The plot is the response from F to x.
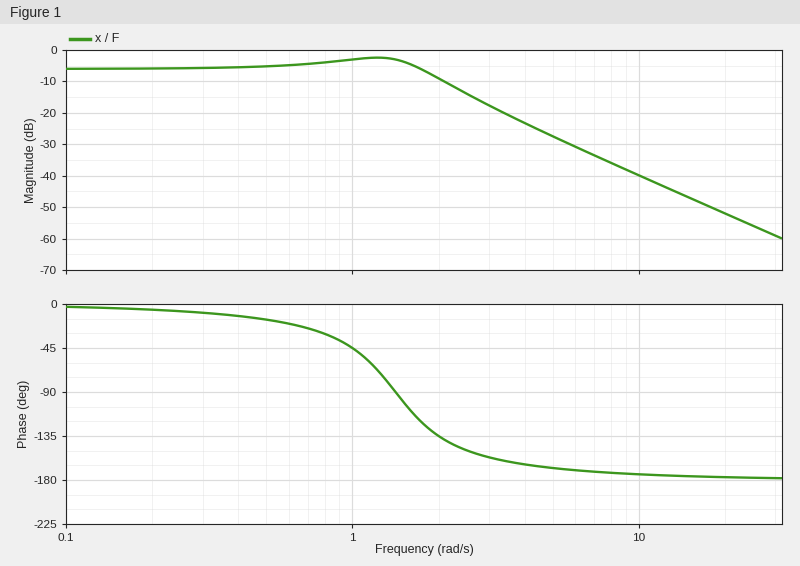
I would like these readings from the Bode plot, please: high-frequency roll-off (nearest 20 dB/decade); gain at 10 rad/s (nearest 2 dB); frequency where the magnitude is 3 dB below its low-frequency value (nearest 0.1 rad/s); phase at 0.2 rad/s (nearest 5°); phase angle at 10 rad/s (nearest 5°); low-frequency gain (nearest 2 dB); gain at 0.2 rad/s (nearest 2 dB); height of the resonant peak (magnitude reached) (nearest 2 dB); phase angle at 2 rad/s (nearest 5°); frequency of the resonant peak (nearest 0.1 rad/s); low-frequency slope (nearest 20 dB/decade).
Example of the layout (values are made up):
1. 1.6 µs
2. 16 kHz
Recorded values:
1. -40 dB/decade
2. -40 dB
3. 2.0 rad/s
4. -5°
5. -175°
6. -6 dB
7. -6 dB
8. -2 dB
9. -135°
10. 1.2 rad/s
11. 0 dB/decade
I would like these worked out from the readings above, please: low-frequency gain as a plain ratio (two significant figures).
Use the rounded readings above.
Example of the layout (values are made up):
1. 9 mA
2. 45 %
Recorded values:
1. 0.50
